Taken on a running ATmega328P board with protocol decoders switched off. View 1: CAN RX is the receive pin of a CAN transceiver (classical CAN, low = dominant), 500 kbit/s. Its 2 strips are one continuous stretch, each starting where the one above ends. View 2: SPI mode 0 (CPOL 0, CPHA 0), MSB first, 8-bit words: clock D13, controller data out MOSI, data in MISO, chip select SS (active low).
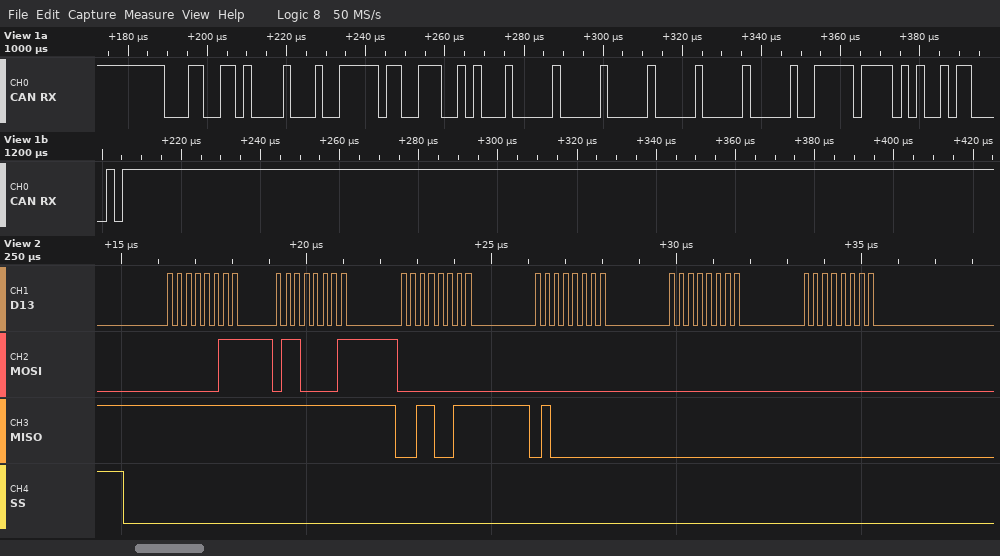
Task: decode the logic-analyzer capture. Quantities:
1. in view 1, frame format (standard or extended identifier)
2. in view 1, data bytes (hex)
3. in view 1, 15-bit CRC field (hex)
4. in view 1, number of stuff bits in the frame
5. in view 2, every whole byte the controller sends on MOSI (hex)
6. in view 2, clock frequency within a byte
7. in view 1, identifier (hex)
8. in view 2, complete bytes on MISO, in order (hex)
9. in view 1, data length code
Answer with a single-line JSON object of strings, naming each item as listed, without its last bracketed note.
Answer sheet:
{"in view 1, frame format": "standard", "in view 1, data bytes": "9F CE 51 00 00 00 00 FF", "in view 1, 15-bit CRC field": "0x54B0", "in view 1, number of stuff bits in the frame": "8", "in view 2, every whole byte the controller sends on MOSI": "03 61 00 00 00 00", "in view 2, clock frequency within a byte": "4 MHz", "in view 1, identifier": "0x19A", "in view 2, complete bytes on MISO, in order": "FF FF 33 40 00 00", "in view 1, data length code": "8"}
